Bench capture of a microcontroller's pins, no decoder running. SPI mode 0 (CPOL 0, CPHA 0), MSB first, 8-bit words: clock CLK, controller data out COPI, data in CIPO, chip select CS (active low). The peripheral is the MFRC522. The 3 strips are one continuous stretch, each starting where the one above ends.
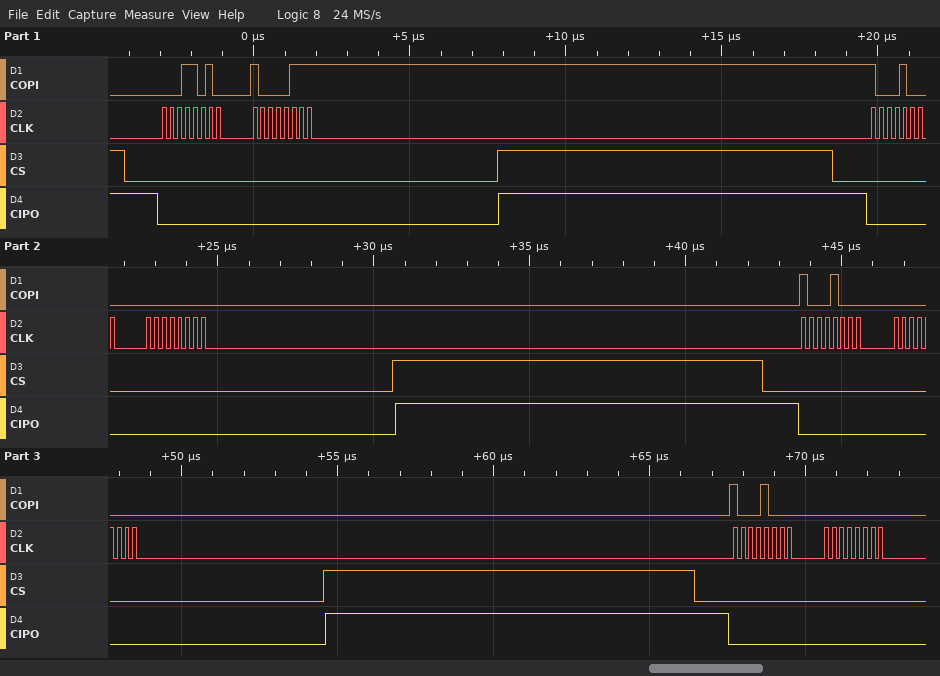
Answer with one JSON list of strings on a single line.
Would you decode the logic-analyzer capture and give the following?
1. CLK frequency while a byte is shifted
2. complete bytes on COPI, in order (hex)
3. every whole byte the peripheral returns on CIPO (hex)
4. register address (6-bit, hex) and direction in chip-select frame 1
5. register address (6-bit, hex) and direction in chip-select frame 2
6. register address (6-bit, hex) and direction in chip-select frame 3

["4 MHz", "1A 87 88 00 88 00 88 00", "00 00 00 00 00 00 00 00", "0x0D write", "0x04 read", "0x04 read"]
